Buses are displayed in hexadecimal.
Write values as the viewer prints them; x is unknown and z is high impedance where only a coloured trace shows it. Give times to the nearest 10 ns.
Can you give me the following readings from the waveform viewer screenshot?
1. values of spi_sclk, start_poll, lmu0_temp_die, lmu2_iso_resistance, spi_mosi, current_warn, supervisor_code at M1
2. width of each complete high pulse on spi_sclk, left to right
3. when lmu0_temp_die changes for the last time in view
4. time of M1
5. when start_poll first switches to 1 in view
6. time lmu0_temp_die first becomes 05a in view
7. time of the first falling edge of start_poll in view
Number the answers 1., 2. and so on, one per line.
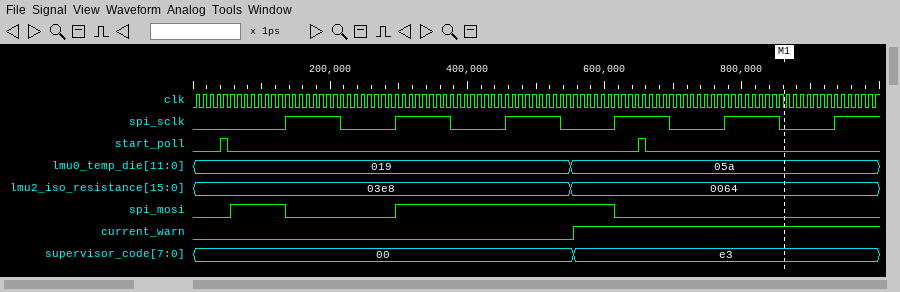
1. spi_sclk=0, start_poll=0, lmu0_temp_die=05a, lmu2_iso_resistance=0064, spi_mosi=0, current_warn=1, supervisor_code=e3
2. 80 ns, 80 ns, 80 ns, 80 ns, 80 ns
3. 550 ns
4. 860 ns
5. 40 ns
6. 550 ns
7. 50 ns
